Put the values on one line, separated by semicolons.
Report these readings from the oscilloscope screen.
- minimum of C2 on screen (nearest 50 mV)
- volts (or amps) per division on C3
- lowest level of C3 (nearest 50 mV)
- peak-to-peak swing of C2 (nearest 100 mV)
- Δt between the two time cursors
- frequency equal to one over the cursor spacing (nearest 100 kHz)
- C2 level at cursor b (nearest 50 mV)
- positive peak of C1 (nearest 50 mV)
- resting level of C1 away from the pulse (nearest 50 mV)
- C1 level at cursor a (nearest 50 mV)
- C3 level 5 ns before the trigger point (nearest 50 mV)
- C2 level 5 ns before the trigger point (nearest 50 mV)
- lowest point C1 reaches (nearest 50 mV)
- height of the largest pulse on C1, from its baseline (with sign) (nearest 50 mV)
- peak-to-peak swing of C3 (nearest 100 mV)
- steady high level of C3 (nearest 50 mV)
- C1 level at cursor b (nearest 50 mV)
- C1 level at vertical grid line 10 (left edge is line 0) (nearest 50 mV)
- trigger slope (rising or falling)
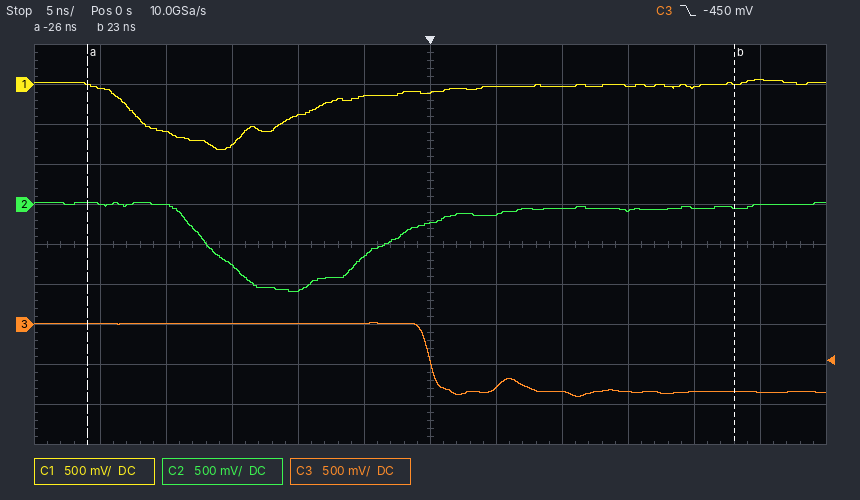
-1.10 V; 500 mV; -900 mV; 1.10 V; 49.0 ns; 20.4 MHz; -50 mV; 50 mV; 0 mV; 0 mV; 0 mV; -650 mV; -800 mV; -800 mV; 900 mV; 0 mV; 0 mV; -50 mV; falling
